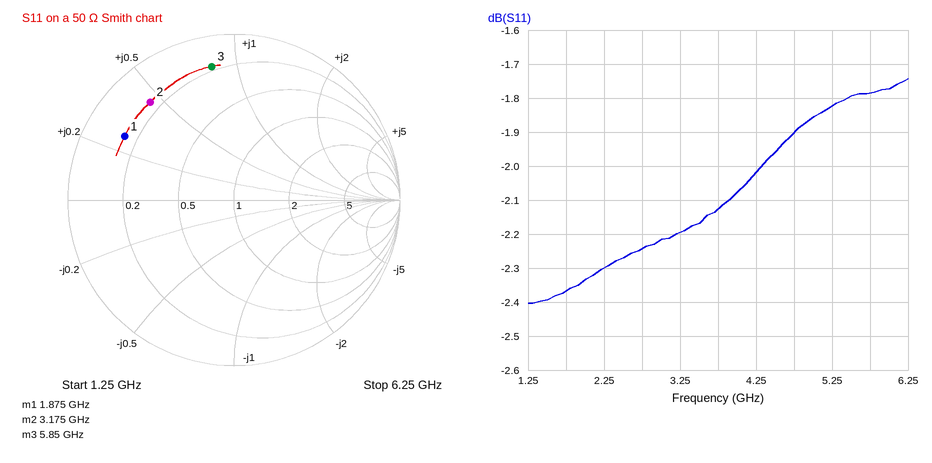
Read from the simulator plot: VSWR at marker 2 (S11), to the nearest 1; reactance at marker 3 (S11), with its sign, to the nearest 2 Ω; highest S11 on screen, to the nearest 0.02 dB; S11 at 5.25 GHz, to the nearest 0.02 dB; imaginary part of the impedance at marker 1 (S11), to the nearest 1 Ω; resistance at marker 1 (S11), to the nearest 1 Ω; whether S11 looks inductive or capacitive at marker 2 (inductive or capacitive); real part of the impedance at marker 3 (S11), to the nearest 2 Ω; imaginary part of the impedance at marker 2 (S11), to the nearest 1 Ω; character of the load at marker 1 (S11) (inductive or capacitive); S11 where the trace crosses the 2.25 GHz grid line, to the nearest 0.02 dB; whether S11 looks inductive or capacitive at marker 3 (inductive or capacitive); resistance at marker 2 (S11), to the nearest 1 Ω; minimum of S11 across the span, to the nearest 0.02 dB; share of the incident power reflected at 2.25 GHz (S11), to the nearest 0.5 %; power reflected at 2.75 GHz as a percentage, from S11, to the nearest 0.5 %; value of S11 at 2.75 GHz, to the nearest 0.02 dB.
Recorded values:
8
+42 Ω
-1.74 dB
-1.82 dB
+13 Ω
7 Ω
inductive
8 Ω
+23 Ω
inductive
-2.30 dB
inductive
8 Ω
-2.40 dB
59.0 %
59.5 %
-2.24 dB
